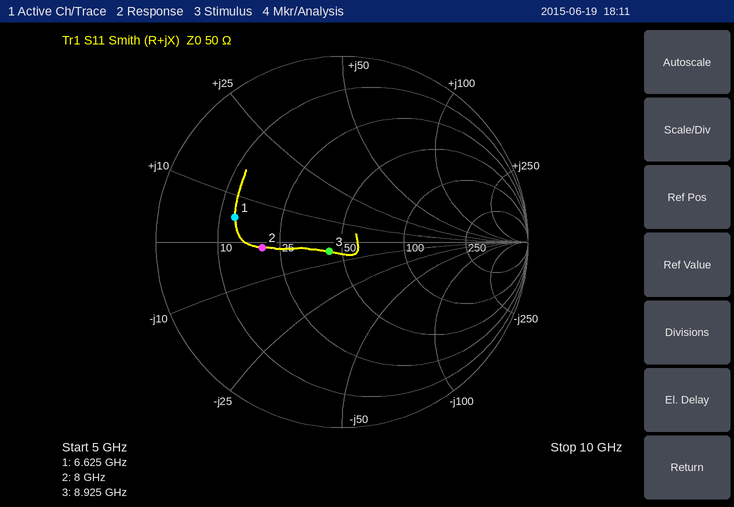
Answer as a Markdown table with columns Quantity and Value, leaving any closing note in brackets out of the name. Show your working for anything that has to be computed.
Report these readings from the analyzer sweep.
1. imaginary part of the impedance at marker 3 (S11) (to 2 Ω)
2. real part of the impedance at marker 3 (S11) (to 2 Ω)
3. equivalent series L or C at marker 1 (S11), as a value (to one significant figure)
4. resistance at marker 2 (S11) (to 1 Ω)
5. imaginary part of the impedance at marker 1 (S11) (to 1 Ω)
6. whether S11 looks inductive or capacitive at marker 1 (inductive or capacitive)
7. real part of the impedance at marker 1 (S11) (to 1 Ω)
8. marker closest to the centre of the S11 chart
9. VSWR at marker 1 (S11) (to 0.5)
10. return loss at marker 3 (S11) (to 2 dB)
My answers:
| Quantity | Value |
|---|---|
| imaginary part of the impedance at marker 3 (S11) | -4 Ω |
| real part of the impedance at marker 3 (S11) | 44 Ω |
| equivalent series L or C at marker 1 (S11), as a value | L = 5 Ω/(2π × 6.625 GHz) ≈ 120 pH, so 100 pH to one significant figure |
| resistance at marker 2 (S11) | 20 Ω |
| imaginary part of the impedance at marker 1 (S11) | +5 Ω |
| whether S11 looks inductive or capacitive at marker 1 | inductive |
| real part of the impedance at marker 1 (S11) | 13 Ω |
| marker closest to the centre of the S11 chart | marker 3 |
| VSWR at marker 1 (S11) | 4.0 |
| return loss at marker 3 (S11) | 22 dB |
